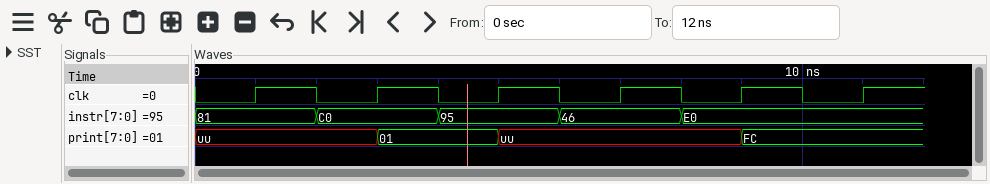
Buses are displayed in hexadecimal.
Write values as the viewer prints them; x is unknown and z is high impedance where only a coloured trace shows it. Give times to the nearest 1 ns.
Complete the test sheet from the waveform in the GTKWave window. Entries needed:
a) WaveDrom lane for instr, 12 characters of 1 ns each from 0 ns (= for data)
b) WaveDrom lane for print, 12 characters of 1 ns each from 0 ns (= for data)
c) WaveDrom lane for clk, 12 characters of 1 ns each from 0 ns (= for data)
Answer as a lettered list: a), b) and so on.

a) {name: 'instr', wave: '=.=.=.=.=...', data: '81 C0 95 46 E0'}
b) {name: 'print', wave: 'x..=.x...=..', data: '01 FC'}
c) {name: 'clk', wave: '010101010101'}
